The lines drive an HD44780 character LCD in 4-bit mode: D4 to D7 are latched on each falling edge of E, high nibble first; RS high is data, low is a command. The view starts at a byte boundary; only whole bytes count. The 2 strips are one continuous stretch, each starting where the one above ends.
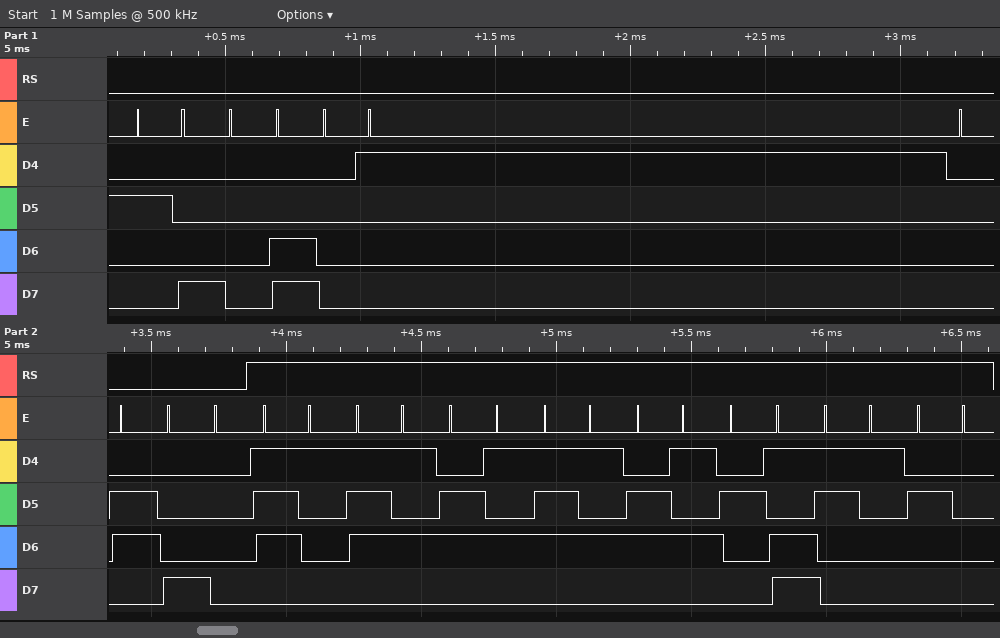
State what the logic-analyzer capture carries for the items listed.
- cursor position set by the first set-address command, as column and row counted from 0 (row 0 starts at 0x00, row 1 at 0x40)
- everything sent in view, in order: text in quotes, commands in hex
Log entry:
column 0, row 0
0x28 0x0C 0x01 0x06 0x80 "queue-1 "
